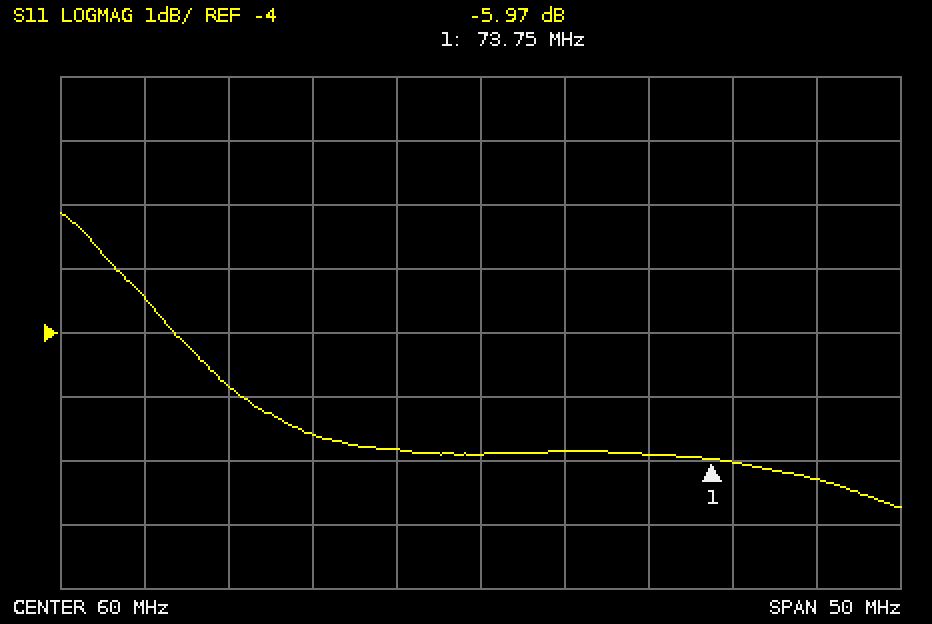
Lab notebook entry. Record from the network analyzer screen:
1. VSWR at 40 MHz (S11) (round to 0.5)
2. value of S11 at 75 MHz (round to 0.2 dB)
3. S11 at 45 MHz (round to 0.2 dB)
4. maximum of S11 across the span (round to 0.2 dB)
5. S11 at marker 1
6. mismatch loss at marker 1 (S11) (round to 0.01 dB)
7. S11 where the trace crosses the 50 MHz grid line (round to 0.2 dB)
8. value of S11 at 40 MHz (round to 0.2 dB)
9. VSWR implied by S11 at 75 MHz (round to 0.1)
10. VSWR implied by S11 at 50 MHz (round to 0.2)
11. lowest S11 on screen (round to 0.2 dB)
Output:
5.0
-6.0 dB
-4.8 dB
-2.2 dB
-5.97 dB
1.27 dB
-5.6 dB
-3.4 dB
3.0
3.2
-6.8 dB
